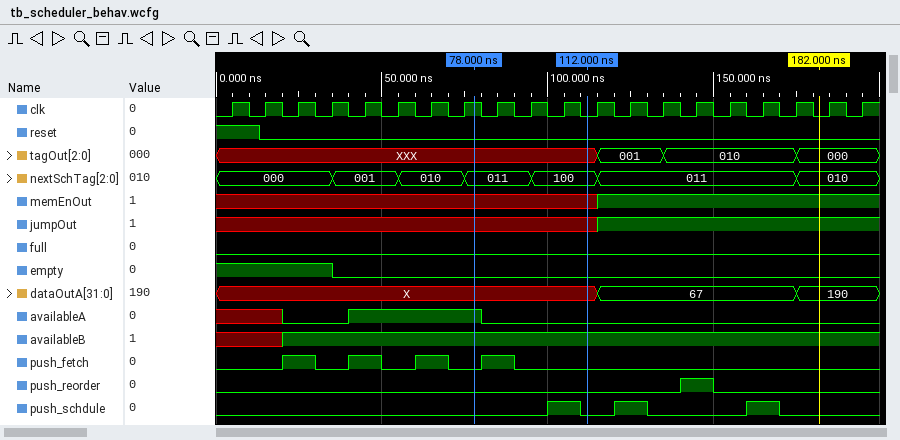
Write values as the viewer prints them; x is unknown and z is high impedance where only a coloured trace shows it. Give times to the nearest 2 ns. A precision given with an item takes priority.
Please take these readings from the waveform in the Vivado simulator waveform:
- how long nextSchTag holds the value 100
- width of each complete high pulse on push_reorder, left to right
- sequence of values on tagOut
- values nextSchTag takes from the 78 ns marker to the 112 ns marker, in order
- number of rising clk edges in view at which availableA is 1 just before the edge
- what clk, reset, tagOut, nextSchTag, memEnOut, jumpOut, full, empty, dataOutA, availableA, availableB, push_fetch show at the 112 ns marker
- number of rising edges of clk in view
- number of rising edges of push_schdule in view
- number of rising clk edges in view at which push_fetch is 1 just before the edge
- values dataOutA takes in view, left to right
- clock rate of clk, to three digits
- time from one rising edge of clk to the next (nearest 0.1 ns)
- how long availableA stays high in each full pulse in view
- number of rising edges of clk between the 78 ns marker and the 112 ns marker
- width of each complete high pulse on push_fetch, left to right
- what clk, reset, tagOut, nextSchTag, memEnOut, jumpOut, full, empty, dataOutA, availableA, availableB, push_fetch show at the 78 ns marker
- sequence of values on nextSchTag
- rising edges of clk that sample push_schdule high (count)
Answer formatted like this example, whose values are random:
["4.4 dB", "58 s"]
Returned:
["20 ns", "10 ns", "XXX, 001, 010, 000", "011, 100", "4", "clk=0, reset=0, tagOut=XXX, nextSchTag=100, memEnOut=x, jumpOut=x, full=0, empty=0, dataOutA=X, availableA=0, availableB=1, push_fetch=0", "20", "3", "4", "X, 67, 190", "100 MHz", "10 ns", "40 ns", "3", "10 ns, 10 ns, 10 ns, 10 ns", "clk=1, reset=0, tagOut=XXX, nextSchTag=011, memEnOut=x, jumpOut=x, full=0, empty=0, dataOutA=X, availableA=1, availableB=1, push_fetch=0", "000, 001, 010, 011, 100, 011, 010", "3"]
